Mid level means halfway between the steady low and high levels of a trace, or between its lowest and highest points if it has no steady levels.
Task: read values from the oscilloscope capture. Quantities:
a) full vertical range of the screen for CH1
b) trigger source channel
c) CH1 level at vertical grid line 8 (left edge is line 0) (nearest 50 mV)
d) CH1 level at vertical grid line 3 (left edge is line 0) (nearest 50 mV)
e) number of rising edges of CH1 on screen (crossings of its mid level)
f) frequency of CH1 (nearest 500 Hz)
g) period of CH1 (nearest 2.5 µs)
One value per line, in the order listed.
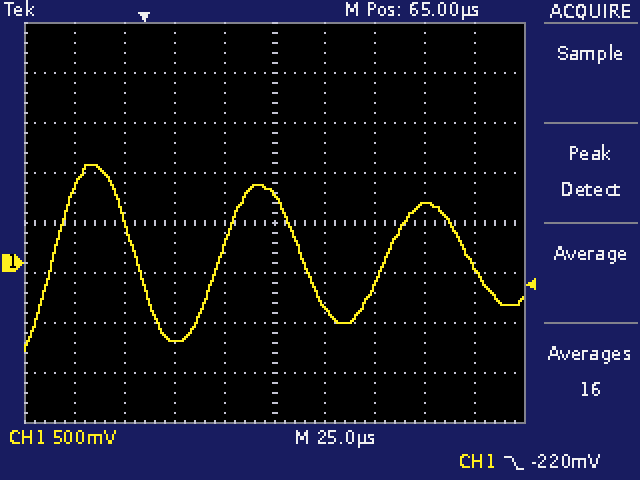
4 V
CH1
600 mV
-800 mV
3
12.0 kHz
82.5 µs
